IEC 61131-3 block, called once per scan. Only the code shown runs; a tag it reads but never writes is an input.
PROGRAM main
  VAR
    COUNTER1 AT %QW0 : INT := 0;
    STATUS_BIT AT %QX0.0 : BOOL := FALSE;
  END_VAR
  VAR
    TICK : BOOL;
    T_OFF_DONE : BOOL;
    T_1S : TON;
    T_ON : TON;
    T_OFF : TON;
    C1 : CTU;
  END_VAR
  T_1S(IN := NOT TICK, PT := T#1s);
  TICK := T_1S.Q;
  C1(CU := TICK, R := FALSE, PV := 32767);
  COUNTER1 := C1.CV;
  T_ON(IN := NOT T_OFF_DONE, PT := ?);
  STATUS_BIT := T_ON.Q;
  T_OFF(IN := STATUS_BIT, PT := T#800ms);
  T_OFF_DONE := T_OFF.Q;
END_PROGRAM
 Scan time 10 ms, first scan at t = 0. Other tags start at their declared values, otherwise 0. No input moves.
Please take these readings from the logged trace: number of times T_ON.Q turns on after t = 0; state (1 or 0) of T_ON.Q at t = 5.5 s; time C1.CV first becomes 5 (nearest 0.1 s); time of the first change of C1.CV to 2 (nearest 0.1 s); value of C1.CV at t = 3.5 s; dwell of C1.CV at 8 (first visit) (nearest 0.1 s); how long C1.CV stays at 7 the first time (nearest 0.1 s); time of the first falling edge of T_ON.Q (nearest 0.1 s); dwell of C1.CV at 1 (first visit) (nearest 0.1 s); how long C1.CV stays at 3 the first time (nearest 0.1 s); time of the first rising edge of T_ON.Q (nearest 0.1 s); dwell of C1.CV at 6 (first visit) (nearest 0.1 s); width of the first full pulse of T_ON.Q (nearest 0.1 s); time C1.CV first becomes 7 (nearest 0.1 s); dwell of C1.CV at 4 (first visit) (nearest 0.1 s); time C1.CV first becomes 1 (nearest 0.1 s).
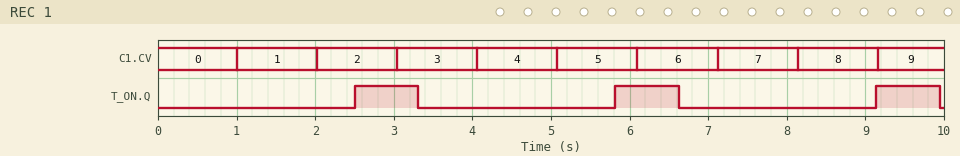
3
0
5.1 s
2.0 s
3
1.0 s
1.0 s
3.3 s
1.0 s
1.0 s
2.5 s
1.0 s
0.8 s
7.1 s
1.0 s
1.0 s
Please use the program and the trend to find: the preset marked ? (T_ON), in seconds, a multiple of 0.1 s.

2.5 s
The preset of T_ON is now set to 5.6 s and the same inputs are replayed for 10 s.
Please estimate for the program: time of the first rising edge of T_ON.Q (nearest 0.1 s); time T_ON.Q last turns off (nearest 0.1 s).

5.6 s
6.4 s
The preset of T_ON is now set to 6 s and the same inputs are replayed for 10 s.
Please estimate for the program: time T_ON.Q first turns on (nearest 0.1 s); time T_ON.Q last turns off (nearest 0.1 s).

6.0 s
6.8 s
